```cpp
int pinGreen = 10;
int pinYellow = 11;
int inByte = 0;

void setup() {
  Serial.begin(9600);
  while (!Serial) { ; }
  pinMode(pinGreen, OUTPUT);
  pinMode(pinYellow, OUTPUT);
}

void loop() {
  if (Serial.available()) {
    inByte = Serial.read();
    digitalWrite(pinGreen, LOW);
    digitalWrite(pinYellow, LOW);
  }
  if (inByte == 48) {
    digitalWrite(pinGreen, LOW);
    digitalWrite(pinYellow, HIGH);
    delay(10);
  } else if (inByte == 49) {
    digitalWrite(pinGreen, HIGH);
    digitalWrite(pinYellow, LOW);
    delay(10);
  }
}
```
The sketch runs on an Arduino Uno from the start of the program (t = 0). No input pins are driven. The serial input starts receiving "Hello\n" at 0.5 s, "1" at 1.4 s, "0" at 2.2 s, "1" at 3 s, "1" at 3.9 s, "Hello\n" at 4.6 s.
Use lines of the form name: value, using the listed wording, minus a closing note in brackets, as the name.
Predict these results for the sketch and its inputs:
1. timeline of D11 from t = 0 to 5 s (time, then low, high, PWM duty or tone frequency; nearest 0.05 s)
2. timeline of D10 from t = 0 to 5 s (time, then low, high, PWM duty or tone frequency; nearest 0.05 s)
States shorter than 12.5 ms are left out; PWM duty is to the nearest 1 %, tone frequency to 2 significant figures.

timeline of D11 from t = 0 to 5 s: 0 s low; 2.2 s high; 3 s low
timeline of D10 from t = 0 to 5 s: 0 s low; 1.4 s high; 2.2 s low; 3 s high; 4.6 s low
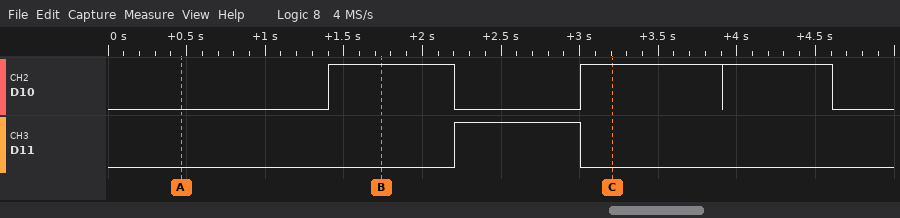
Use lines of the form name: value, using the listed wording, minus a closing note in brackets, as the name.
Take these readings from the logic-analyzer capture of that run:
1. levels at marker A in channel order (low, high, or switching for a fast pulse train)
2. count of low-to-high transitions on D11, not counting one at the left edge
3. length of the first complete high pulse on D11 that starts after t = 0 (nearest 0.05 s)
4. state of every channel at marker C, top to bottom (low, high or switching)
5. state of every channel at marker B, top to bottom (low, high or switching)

levels at marker A in channel order: D10 low, D11 low
count of low-to-high transitions on D11, not counting one at the left edge: 1
length of the first complete high pulse on D11 that starts after t = 0: 0.80 s
state of every channel at marker C, top to bottom: D10 high, D11 low
state of every channel at marker B, top to bottom: D10 high, D11 low
